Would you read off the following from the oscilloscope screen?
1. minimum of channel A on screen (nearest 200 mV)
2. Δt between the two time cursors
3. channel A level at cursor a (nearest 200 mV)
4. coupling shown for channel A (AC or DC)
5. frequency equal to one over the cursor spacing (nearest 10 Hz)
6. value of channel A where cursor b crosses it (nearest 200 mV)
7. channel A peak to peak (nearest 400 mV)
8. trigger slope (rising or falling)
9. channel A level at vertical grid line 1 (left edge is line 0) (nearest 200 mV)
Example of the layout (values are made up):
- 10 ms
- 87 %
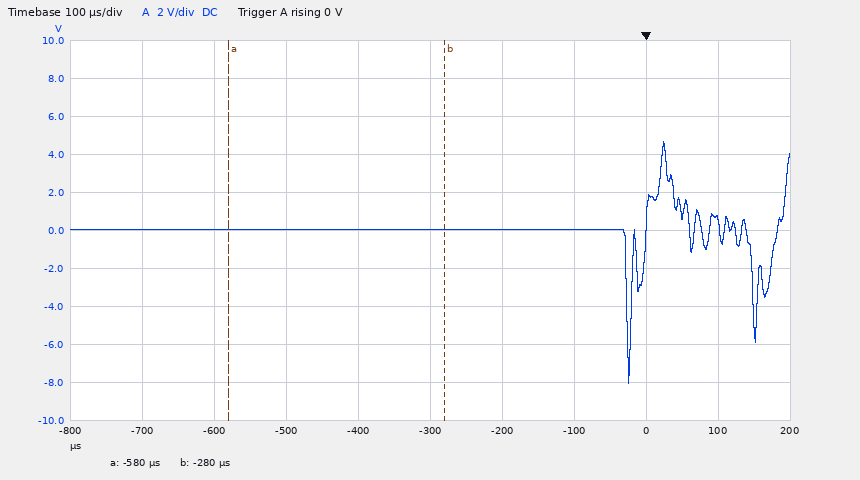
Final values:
- -8.0 V
- 300 µs
- 0.0 V
- DC
- 3.33 kHz
- 0.0 V
- 12.8 V
- rising
- 0.0 V
